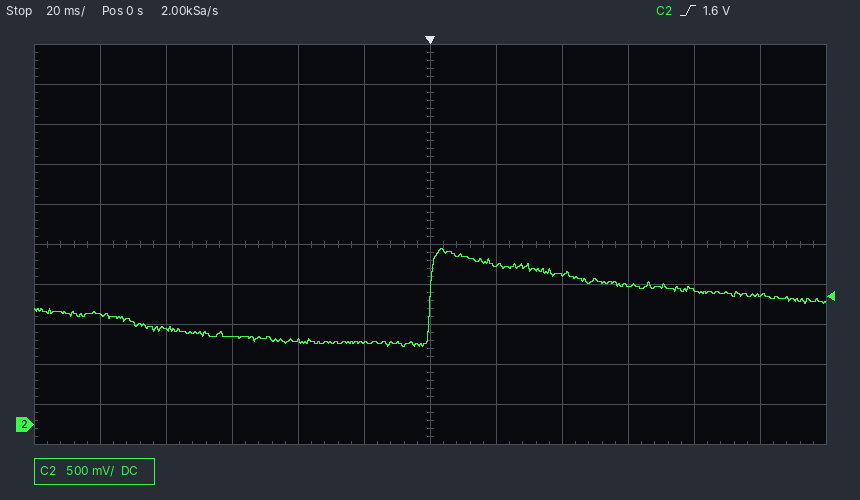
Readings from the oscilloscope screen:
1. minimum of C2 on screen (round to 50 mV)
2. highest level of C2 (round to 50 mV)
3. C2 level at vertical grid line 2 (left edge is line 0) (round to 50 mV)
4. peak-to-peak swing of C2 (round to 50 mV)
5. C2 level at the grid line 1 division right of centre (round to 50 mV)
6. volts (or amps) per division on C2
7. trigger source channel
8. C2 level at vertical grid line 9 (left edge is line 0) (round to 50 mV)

1.00 V
2.20 V
1.20 V
1.20 V
2.00 V
500 mV
C2
1.75 V
